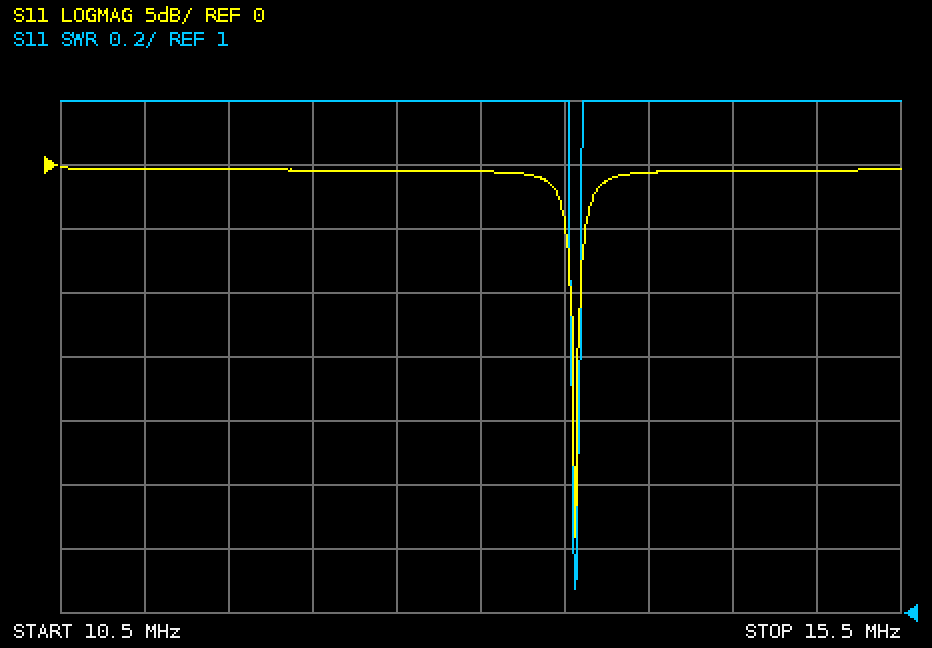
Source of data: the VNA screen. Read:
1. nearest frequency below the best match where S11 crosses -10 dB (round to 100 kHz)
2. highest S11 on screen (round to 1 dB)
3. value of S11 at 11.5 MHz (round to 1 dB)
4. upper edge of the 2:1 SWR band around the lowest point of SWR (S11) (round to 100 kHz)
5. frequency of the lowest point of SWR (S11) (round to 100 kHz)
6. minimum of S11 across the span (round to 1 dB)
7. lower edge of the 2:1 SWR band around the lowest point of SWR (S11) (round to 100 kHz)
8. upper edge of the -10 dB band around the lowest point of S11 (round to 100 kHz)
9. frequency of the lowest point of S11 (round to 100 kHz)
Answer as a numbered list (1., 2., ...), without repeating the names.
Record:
1. 13.5 MHz
2. 0 dB
3. 0 dB
4. 13.6 MHz
5. 13.6 MHz
6. -29 dB
7. 13.5 MHz
8. 13.6 MHz
9. 13.6 MHz
